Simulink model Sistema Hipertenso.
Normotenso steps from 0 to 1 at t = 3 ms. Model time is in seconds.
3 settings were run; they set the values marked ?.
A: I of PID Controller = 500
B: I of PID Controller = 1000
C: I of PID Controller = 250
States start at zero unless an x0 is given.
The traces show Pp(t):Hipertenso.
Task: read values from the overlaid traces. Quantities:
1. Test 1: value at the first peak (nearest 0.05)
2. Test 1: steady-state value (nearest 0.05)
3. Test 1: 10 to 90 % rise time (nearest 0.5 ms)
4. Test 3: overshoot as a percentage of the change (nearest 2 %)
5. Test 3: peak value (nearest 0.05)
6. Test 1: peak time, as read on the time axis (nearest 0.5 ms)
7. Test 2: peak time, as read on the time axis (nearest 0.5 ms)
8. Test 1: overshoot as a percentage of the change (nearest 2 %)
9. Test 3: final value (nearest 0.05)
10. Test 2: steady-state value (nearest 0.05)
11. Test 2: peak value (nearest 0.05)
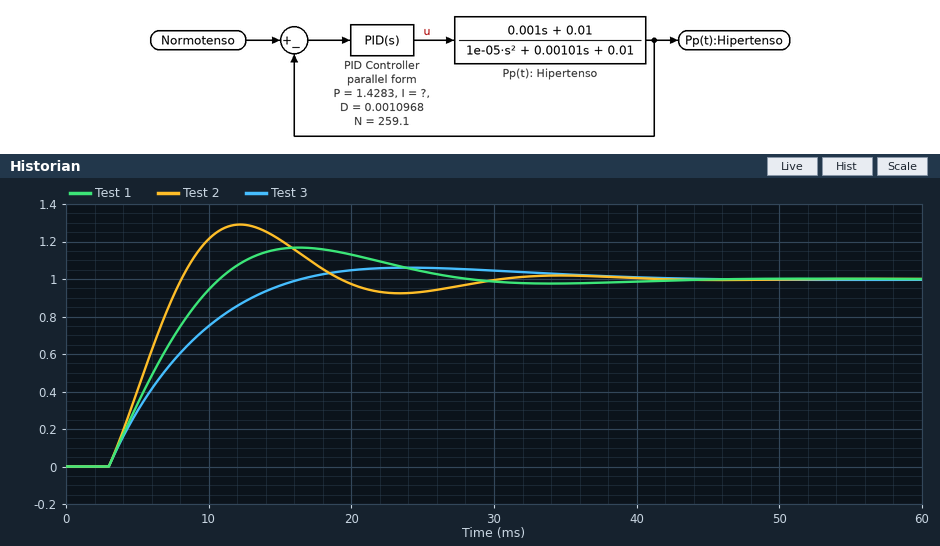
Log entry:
1.15
1.00
6.0 ms
6 %
1.05
16.5 ms
12.0 ms
16 %
1.00
1.00
1.30
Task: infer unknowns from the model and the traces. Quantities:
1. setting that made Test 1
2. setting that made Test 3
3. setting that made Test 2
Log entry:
A
C
B
